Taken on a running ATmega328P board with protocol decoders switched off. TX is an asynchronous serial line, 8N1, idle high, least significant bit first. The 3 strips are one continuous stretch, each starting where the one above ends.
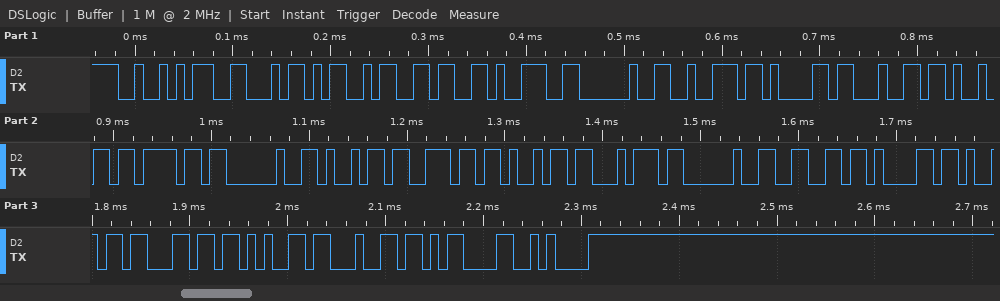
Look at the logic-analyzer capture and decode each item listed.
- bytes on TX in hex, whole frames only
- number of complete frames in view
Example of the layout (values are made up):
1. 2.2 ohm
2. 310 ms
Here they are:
1. 0x52 0x46 0x4D 0x36 0x39 0x20 0x72 0x61 0x64 0x69 0x6F 0x20 0x69 0x6E 0x69 0x74 0x20 0x66 0x61 0x69 0x6C 0x65 0x64 0x0D 0x0A
2. 25
